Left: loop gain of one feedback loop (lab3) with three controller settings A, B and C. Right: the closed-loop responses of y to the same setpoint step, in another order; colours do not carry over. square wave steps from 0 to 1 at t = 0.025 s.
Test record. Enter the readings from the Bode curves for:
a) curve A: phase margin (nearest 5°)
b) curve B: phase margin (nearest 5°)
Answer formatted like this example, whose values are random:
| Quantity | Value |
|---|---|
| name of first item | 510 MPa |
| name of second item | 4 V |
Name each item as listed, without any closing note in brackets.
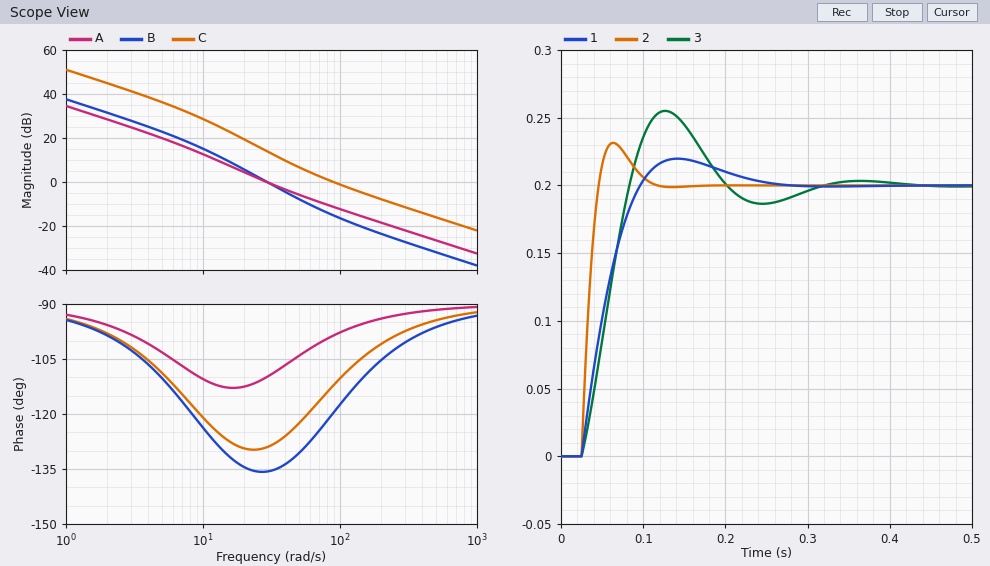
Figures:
| Quantity | Value |
|---|---|
| curve A: phase margin | 70° |
| curve B: phase margin | 45° |
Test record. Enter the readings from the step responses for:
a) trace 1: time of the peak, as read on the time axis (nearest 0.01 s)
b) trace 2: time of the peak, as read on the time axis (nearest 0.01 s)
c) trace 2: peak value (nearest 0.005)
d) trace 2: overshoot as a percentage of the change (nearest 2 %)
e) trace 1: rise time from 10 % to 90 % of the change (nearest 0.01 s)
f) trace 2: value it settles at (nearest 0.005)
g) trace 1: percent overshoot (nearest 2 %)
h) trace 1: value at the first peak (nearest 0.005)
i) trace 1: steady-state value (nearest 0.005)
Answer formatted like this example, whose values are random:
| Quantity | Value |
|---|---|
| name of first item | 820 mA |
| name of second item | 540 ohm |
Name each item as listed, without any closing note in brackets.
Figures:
| Quantity | Value |
|---|---|
| trace 1: time of the peak, as read on the time axis | 0.14 s |
| trace 2: time of the peak, as read on the time axis | 0.06 s |
| trace 2: peak value | 0.230 |
| trace 2: overshoot as a percentage of the change | 16 % |
| trace 1: rise time from 10 % to 90 % of the change | 0.05 s |
| trace 2: value it settles at | 0.200 |
| trace 1: percent overshoot | 10 % |
| trace 1: value at the first peak | 0.220 |
| trace 1: steady-state value | 0.200 |
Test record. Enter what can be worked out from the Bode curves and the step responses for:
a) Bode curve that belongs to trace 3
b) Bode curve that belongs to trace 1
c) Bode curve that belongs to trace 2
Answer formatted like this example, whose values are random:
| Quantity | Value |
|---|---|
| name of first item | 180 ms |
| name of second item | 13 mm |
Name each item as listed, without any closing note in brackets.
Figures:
| Quantity | Value |
|---|---|
| Bode curve that belongs to trace 3 | B |
| Bode curve that belongs to trace 1 | A |
| Bode curve that belongs to trace 2 | C |
